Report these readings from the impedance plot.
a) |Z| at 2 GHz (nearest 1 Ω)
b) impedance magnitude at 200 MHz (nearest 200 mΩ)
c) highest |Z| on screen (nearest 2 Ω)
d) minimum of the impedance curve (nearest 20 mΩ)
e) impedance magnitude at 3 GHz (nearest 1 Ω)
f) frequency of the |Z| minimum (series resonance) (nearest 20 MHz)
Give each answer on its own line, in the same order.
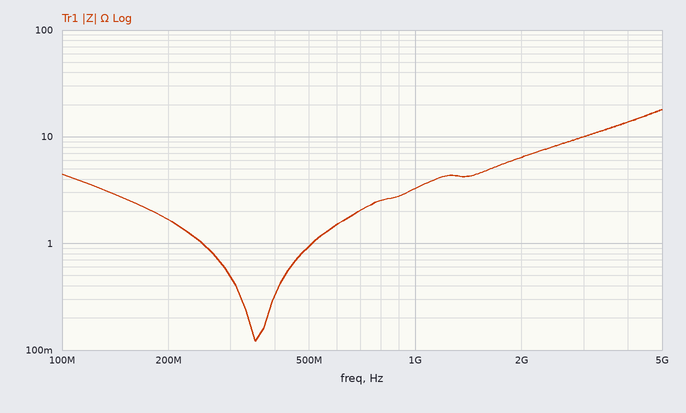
6 Ω
1.6 Ω
18 Ω
120 mΩ
10 Ω
360 MHz
